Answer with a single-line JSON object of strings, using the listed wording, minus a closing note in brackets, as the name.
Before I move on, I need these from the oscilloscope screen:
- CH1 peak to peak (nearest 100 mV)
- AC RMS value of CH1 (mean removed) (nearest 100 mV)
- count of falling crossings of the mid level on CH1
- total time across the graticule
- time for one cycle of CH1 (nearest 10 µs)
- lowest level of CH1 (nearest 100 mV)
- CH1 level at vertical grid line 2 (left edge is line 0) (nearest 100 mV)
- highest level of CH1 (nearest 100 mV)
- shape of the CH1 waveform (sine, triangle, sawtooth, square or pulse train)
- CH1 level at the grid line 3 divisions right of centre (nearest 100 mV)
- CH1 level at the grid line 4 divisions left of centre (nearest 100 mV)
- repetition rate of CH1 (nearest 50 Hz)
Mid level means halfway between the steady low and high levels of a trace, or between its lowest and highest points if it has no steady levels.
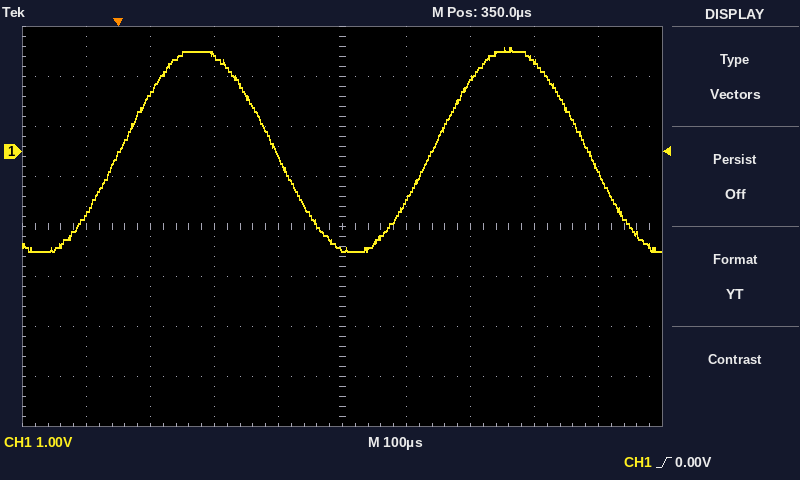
{"CH1 peak to peak": "4.1 V", "AC RMS value of CH1 (mean removed)": "1.4 V", "count of falling crossings of the mid level on CH1": "2", "total time across the graticule": "1 ms", "time for one cycle of CH1": "490 µs", "lowest level of CH1": "-2.0 V", "CH1 level at vertical grid line 2 (left edge is line 0)": "1.1 V", "highest level of CH1": "2.1 V", "shape of the CH1 waveform": "sine", "CH1 level at the grid line 3 divisions right of centre": "1.8 V", "CH1 level at the grid line 4 divisions left of centre": "-1.3 V", "repetition rate of CH1": "2.05 kHz"}
